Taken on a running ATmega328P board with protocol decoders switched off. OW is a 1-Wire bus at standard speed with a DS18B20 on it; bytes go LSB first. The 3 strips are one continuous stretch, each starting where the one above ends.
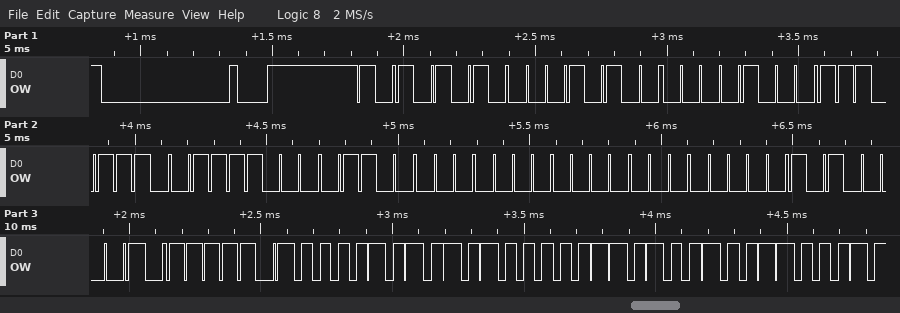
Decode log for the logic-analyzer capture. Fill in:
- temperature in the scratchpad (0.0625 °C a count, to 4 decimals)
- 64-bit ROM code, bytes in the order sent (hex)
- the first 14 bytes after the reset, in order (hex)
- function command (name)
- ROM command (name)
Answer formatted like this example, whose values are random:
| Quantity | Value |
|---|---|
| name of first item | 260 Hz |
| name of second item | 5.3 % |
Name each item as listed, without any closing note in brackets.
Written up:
| Quantity | Value |
|---|---|
| temperature in the scratchpad | 85.0000 °C |
| 64-bit ROM code, bytes in the order sent | 28 10 77 1E 06 00 00 85 |
| the first 14 bytes after the reset, in order | 55 28 10 77 1E 06 00 00 85 BE 50 05 4B 46 |
| function command | Read Scratchpad |
| ROM command | Match ROM |
